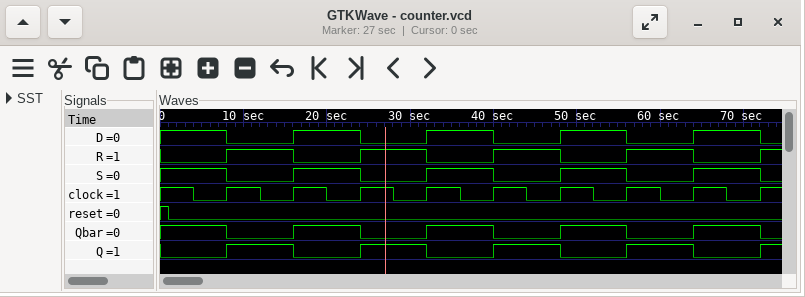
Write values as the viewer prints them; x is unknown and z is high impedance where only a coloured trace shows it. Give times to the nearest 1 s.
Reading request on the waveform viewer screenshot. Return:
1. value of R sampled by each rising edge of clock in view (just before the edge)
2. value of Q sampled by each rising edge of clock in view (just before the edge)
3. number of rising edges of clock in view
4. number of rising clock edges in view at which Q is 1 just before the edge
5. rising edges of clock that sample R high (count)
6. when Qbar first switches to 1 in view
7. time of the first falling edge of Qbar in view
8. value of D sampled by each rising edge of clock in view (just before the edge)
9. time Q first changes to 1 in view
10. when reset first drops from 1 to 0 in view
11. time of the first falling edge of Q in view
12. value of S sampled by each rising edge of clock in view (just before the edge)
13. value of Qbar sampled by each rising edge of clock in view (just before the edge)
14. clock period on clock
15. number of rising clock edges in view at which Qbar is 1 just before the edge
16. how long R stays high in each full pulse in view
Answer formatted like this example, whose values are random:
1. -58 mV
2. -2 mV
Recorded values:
1. 0 1 0 1 0 1 0 1 0
2. 0 1 0 1 0 1 0 1 0
3. 9
4. 4
5. 4
6. 16 s
7. 8 s
8. 1 0 1 0 1 0 1 0 1
9. 8 s
10. 1 s
11. 16 s
12. 1 0 1 0 1 0 1 0 1
13. 1 0 1 0 1 0 1 0 1
14. 8 s
15. 5
16. 8 s, 8 s, 8 s, 8 s
